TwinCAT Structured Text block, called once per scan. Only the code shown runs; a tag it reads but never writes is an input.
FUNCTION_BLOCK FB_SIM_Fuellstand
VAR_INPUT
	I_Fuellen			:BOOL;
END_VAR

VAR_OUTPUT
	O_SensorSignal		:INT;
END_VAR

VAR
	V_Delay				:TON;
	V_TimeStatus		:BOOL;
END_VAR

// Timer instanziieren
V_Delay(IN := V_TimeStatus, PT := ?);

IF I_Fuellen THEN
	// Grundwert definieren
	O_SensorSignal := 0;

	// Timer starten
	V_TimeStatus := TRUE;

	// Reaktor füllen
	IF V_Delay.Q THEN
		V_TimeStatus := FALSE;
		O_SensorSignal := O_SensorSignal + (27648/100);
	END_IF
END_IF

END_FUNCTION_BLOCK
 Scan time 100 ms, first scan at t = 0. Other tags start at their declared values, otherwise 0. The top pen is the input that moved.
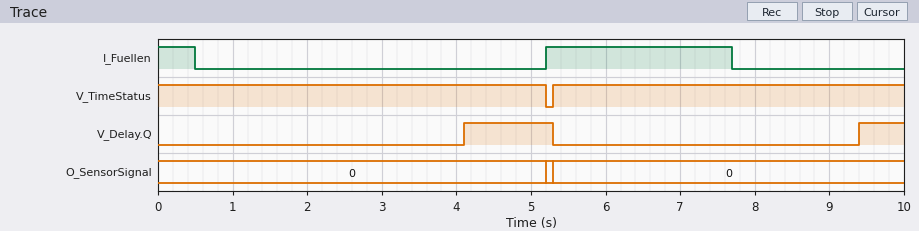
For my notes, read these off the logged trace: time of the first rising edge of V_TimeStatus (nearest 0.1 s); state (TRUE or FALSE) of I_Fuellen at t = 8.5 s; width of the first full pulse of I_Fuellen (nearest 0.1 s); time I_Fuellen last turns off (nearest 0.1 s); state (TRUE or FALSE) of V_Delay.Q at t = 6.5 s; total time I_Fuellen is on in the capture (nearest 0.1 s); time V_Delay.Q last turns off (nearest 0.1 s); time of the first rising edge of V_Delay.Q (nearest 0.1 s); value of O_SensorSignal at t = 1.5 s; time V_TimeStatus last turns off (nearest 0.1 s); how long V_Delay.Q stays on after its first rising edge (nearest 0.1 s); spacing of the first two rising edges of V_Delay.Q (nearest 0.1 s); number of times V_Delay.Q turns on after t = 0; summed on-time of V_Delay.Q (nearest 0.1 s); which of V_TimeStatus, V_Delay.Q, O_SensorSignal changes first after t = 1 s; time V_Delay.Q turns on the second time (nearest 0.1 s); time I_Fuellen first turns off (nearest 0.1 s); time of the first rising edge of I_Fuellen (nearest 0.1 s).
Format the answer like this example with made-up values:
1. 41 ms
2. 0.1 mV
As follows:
1. 5.3 s
2. FALSE
3. 2.5 s
4. 7.7 s
5. FALSE
6. 3.0 s
7. 5.3 s
8. 4.1 s
9. 0
10. 5.2 s
11. 1.2 s
12. 5.3 s
13. 2
14. 1.8 s
15. V_Delay.Q
16. 9.4 s
17. 0.5 s
18. 5.2 s
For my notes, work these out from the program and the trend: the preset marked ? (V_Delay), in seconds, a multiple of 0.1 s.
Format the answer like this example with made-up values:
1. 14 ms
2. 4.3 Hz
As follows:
1. 4.0 s
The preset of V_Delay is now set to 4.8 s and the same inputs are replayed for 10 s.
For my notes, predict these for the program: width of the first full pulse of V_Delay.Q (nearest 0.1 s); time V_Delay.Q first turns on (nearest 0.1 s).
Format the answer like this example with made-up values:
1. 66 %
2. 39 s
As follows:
1. 0.4 s
2. 4.9 s
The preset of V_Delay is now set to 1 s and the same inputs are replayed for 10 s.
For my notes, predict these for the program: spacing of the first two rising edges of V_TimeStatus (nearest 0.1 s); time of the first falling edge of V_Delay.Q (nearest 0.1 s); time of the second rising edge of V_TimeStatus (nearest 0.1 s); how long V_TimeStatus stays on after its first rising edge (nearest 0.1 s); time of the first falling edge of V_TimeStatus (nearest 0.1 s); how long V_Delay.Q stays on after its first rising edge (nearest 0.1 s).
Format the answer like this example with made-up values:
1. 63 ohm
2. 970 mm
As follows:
1. 1.2 s
2. 5.3 s
3. 6.5 s
4. 1.1 s
5. 5.2 s
6. 4.2 s
